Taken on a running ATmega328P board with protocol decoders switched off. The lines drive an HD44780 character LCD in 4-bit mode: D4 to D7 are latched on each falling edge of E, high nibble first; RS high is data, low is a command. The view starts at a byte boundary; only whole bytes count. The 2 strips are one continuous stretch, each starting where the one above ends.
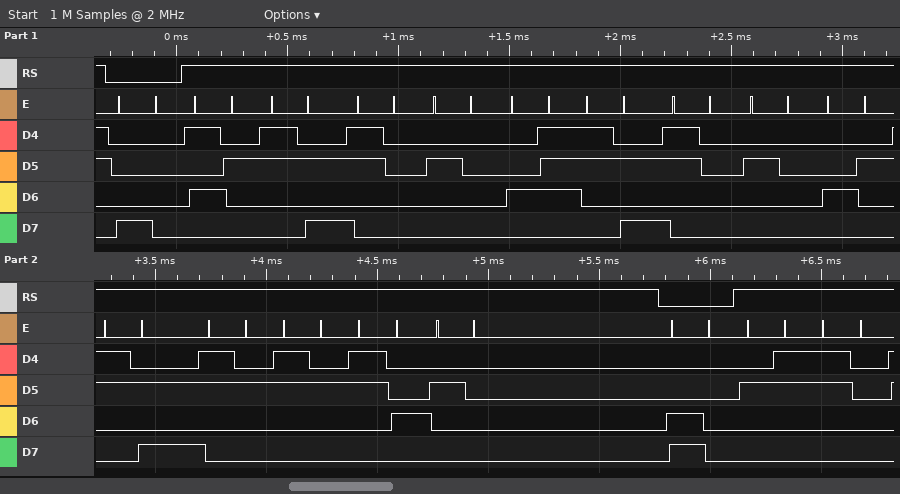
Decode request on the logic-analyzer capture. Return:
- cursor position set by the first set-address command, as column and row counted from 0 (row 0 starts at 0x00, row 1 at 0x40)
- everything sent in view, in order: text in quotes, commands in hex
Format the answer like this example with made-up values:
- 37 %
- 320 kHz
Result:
- column 0, row 0
- 0x80 "R:0 G:0 B:224 " 0xC0 "#0"
